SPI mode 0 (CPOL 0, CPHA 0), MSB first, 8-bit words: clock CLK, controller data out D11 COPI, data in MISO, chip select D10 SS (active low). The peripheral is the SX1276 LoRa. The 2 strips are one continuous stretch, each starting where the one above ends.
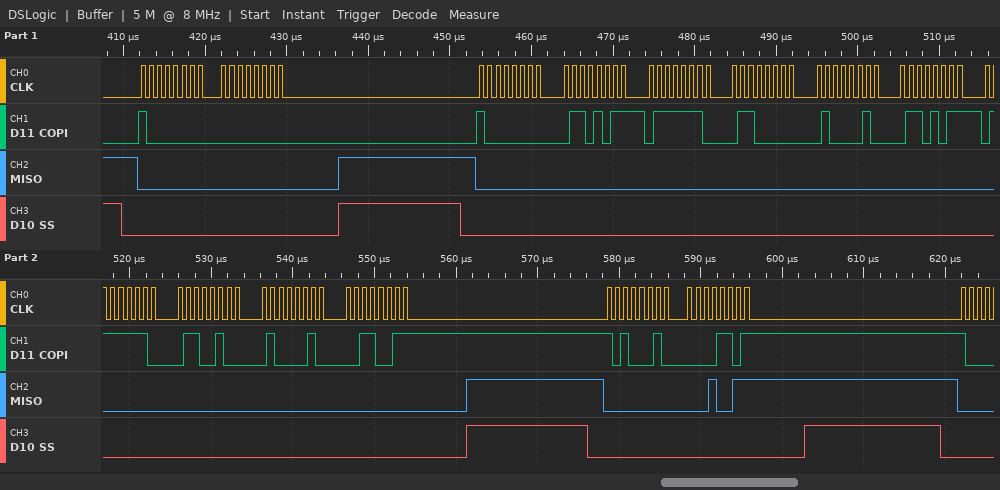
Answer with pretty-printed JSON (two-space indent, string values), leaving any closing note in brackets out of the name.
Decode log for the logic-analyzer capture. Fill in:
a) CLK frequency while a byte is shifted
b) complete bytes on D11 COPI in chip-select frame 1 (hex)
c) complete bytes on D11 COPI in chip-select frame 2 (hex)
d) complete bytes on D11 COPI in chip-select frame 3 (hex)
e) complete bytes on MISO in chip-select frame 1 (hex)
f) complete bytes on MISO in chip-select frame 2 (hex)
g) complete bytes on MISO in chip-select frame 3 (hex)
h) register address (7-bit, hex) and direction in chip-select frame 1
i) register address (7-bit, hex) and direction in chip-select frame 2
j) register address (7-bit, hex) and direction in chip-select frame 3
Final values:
{
  "CLK frequency while a byte is shifted": "1 MHz",
  "complete bytes on D11 COPI in chip-select frame 1": "80 00",
  "complete bytes on D11 COPI in chip-select frame 2": "80 6B 7E 60 42 6B 7E 64 42 33",
  "complete bytes on D11 COPI in chip-select frame 3": "A2 0D",
  "complete bytes on MISO in chip-select frame 1": "00 00",
  "complete bytes on MISO in chip-select frame 2": "00 00 00 00 00 00 00 00 00 00",
  "complete bytes on MISO in chip-select frame 3": "00 13",
  "register address (7-bit, hex) and direction in chip-select frame 1": "0x00 write",
  "register address (7-bit, hex) and direction in chip-select frame 2": "0x00 write",
  "register address (7-bit, hex) and direction in chip-select frame 3": "0x22 write"
}
